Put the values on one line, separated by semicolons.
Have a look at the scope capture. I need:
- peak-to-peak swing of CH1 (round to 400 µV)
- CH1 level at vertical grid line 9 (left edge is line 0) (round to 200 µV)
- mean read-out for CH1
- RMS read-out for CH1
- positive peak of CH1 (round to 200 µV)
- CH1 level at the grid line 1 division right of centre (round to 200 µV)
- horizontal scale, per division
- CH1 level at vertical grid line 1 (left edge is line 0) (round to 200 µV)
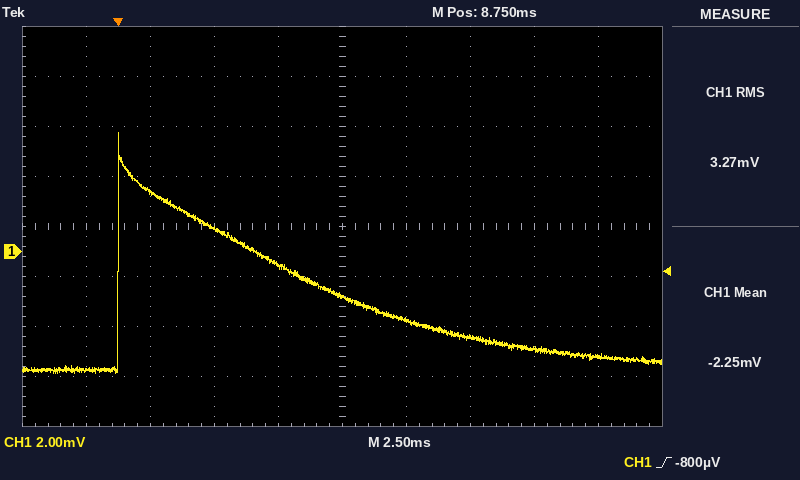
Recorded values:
9.6 mV; -4.2 mV; -2.25 mV; 3.27 mV; 4.8 mV; -2.8 mV; 2.5 ms; -4.8 mV
